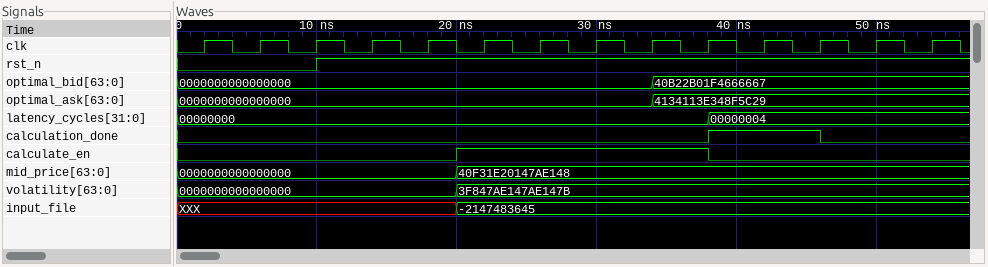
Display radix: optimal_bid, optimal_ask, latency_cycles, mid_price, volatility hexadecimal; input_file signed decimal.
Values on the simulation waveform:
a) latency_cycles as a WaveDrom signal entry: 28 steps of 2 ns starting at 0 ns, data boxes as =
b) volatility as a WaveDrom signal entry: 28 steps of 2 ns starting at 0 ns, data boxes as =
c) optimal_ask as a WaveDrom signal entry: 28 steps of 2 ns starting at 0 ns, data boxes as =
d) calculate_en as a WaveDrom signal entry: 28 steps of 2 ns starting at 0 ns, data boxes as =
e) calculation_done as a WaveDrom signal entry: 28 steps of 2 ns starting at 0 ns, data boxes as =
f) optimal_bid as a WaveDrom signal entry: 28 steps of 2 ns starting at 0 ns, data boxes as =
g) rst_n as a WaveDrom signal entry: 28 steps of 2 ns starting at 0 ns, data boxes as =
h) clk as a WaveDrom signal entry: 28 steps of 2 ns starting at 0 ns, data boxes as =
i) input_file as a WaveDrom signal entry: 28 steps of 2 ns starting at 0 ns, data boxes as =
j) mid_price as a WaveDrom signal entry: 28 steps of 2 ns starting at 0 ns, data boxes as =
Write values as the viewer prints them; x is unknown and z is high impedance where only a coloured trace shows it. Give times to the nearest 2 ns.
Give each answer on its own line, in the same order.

{name: 'latency_cycles', wave: '=..................=........', data: '00000000 00000004'}
{name: 'volatility', wave: '=.........=.................', data: '0000000000000000 3F847AE147AE147B'}
{name: 'optimal_ask', wave: '=................=..........', data: '0000000000000000 4134113E348F5C29'}
{name: 'calculate_en', wave: '0.........1........0........'}
{name: 'calculation_done', wave: '0..................1...0....'}
{name: 'optimal_bid', wave: '=................=..........', data: '0000000000000000 40B22B01F4666667'}
{name: 'rst_n', wave: '0....1......................'}
{name: 'clk', wave: '0101010101010101010101010101'}
{name: 'input_file', wave: 'x.........=.................', data: '-2147483645'}
{name: 'mid_price', wave: '=.........=.................', data: '0000000000000000 40F31E20147AE148'}
